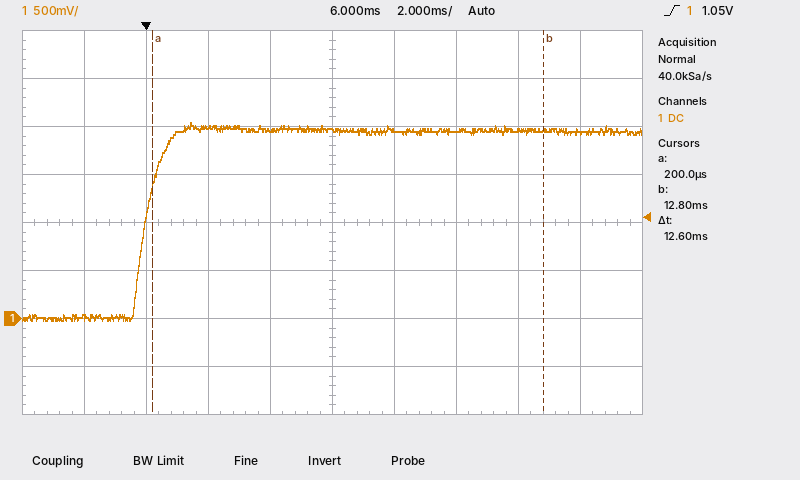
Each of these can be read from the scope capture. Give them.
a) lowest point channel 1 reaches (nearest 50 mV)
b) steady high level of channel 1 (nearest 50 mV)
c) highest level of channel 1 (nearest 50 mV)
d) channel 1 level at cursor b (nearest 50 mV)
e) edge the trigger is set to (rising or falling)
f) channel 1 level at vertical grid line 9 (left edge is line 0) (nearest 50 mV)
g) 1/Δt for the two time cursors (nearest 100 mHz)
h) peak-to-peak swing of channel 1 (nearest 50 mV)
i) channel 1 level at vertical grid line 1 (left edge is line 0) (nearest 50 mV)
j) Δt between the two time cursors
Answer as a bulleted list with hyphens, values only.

- 0 mV
- 1.95 V
- 2.05 V
- 1.95 V
- rising
- 1.95 V
- 79.4 Hz
- 2.05 V
- 0 mV
- 12.6 ms
